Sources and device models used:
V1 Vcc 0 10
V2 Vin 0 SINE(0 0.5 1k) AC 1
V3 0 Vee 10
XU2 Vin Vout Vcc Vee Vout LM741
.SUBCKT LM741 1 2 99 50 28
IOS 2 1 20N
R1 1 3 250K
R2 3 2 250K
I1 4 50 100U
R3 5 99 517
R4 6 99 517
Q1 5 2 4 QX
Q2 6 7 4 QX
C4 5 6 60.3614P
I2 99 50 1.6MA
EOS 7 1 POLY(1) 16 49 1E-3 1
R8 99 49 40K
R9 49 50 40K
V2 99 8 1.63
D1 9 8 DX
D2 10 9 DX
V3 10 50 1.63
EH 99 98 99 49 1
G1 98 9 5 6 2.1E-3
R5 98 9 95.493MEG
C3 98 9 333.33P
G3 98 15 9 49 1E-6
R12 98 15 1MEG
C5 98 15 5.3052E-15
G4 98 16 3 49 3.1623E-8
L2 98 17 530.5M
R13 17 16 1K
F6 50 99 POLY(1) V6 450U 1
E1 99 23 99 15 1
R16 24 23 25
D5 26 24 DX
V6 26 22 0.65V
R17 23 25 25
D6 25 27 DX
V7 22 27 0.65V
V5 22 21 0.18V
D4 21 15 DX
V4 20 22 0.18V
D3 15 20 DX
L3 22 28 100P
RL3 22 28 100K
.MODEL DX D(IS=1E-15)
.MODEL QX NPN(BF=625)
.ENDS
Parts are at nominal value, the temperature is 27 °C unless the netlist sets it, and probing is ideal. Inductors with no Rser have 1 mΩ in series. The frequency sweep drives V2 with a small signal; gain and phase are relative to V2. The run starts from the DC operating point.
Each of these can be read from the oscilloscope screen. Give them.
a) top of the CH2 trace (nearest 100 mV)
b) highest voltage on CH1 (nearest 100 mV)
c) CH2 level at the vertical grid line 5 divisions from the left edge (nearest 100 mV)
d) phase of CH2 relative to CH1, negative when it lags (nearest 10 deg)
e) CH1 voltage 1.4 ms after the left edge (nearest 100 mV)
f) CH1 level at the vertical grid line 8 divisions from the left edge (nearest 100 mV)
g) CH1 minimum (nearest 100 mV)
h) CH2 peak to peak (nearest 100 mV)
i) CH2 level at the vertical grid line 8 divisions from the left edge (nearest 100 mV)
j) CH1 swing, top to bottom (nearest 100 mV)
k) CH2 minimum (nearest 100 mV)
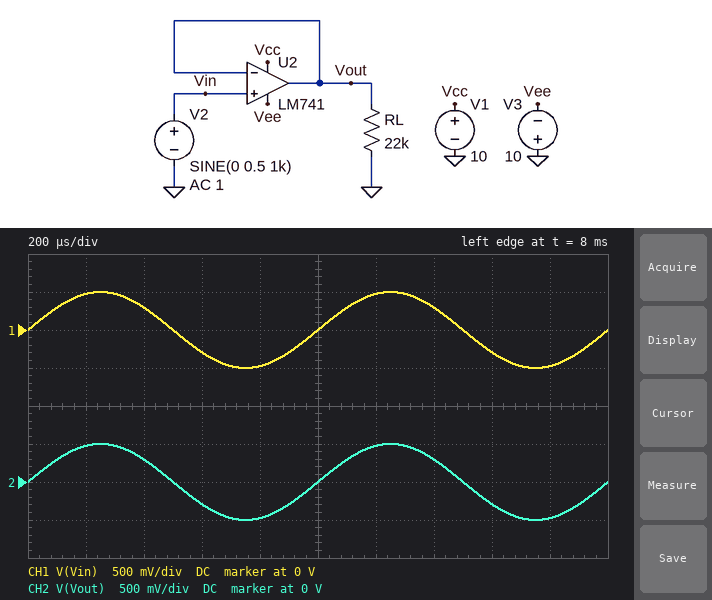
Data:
500 mV
500 mV
0 V
0 deg
300 mV
-300 mV
-500 mV
1.0 V
-300 mV
1.0 V
-500 mV
